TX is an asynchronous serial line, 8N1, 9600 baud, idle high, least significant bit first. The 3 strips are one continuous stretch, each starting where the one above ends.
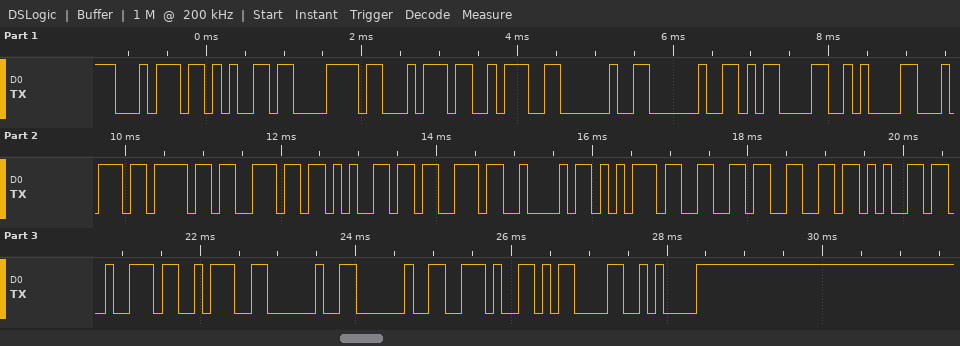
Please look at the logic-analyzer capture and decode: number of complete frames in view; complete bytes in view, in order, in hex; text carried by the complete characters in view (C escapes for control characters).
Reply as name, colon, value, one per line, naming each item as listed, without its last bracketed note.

number of complete frames in view: 26
complete bytes in view, in order, in hex: 74 65 78 74 3A 20 20 0D 0A 74 6F 6E 65 73 42 75 66 66 65 72 3A 20 20 2E 0D 0A
text carried by the complete characters in view: "text:  \r\ntonesBuffer:  .\r\n"
